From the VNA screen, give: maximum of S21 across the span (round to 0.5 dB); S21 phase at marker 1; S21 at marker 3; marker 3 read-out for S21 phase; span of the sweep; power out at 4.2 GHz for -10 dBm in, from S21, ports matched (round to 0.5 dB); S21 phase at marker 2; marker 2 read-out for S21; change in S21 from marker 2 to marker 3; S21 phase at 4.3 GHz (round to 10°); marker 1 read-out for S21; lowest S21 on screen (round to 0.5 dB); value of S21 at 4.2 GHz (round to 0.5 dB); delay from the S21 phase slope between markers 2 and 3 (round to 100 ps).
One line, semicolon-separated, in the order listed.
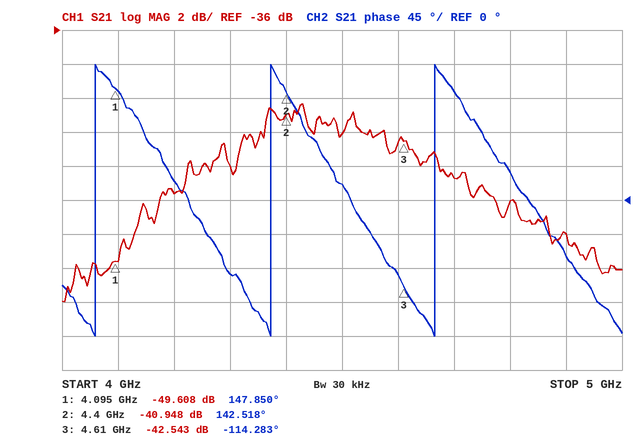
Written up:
-40.5 dB; 147.850°; -42.543 dB; -114.283°; 1 GHz; -55.5 dBm; 142.518°; -40.948 dB; -1.595 dB; -100°; -49.608 dB; -52.0 dB; -45.5 dB; 3.4 ns
